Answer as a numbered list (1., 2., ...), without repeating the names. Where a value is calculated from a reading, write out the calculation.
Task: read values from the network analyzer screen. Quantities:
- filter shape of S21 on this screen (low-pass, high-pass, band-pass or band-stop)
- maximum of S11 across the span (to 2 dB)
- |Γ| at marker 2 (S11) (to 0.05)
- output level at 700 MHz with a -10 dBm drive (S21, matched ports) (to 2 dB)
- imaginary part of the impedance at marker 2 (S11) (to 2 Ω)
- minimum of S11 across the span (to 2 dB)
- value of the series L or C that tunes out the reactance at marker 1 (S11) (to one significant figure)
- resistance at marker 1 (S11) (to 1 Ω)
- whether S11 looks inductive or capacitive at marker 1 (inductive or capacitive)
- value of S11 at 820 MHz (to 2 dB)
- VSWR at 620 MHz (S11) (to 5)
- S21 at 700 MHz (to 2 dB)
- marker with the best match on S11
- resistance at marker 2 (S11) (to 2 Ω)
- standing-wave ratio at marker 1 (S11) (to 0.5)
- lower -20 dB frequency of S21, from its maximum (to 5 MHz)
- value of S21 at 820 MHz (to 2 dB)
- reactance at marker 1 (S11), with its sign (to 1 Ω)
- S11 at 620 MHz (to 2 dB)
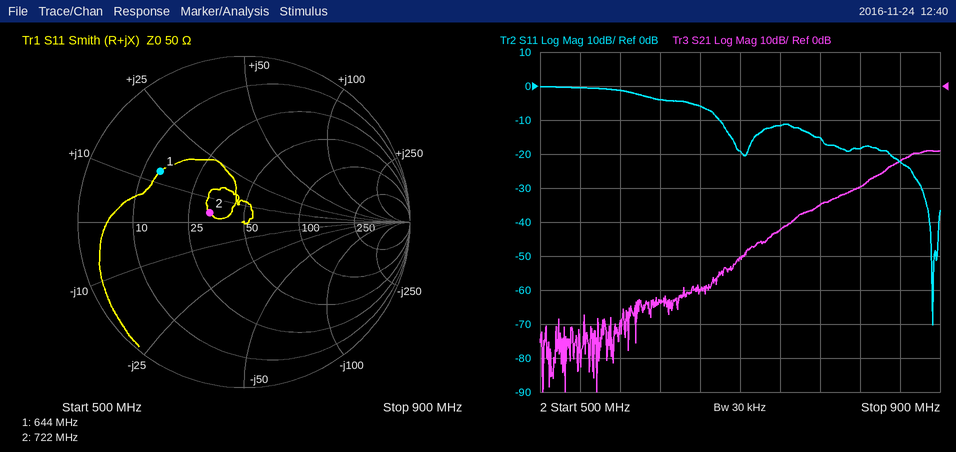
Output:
1. high-pass
2. 0 dB
3. 0.20
4. -10 dBm + (-50 dB) = -60 dBm
5. +4 Ω
6. -70 dB
7. C = 1/(2π × 644 MHz × 13 Ω) ≈ 19.0 pF, so 20 pF to one significant figure
8. 14 Ω
9. inductive
10. -18 dB
11. |Γ| = 10^(-4/20) = 0.6310; VSWR = (1 + 0.6310)/(1 − 0.6310) ≈ 4.42, so 5 to the nearest 5
12. -50 dB
13. marker 2
14. 32 Ω
15. 4.0
16. 755 MHz
17. -30 dB
18. +13 Ω
19. -4 dB
